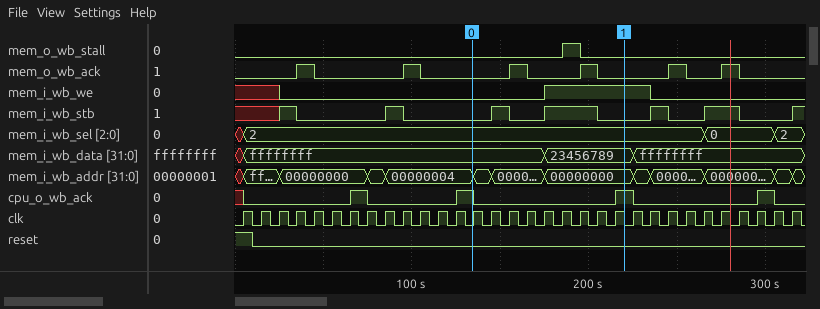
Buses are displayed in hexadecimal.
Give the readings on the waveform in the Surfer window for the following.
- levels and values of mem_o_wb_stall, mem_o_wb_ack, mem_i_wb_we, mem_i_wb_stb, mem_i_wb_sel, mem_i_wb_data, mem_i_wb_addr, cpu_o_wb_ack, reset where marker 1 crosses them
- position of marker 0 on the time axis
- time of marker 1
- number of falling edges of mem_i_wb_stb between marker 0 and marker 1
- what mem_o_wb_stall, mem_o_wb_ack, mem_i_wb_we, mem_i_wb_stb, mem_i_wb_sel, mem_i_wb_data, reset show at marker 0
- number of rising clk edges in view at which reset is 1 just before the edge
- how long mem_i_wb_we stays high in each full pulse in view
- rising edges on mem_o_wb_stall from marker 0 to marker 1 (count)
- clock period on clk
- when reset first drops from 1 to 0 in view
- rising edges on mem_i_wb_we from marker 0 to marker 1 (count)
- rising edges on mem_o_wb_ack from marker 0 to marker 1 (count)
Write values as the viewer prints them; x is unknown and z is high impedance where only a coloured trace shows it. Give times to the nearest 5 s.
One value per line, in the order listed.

mem_o_wb_stall=0, mem_o_wb_ack=0, mem_i_wb_we=1, mem_i_wb_stb=0, mem_i_wb_sel=2, mem_i_wb_data=23456789, mem_i_wb_addr=00000000, cpu_o_wb_ack=1, reset=0
135 s
220 s
2
mem_o_wb_stall=0, mem_o_wb_ack=0, mem_i_wb_we=0, mem_i_wb_stb=0, mem_i_wb_sel=2, mem_i_wb_data=ffffffff, reset=0
1
60 s
1
10 s
10 s
1
2
